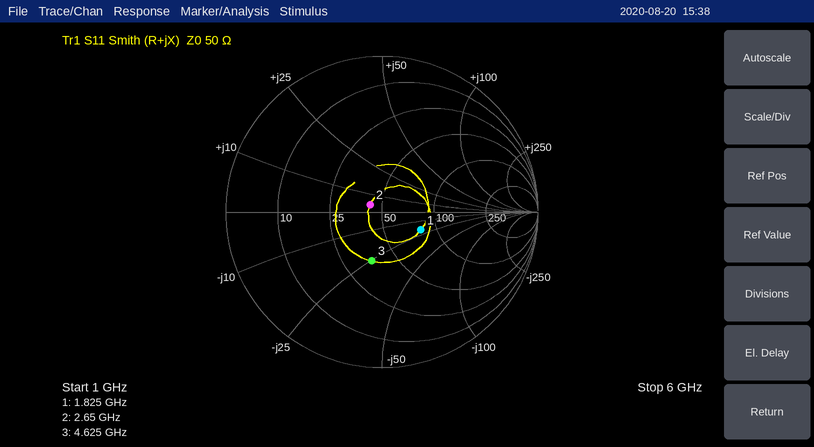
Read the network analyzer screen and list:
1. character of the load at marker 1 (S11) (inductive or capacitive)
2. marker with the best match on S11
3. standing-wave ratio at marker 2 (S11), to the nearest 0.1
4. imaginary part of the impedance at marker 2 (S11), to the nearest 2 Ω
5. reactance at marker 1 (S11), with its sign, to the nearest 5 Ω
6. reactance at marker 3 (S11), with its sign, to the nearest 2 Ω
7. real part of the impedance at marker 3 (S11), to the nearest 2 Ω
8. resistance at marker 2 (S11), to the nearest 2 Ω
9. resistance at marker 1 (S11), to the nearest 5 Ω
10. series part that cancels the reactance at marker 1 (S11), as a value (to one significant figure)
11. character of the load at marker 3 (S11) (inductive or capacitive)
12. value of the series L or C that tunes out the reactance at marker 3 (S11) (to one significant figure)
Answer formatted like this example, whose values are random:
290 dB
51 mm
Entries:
capacitive
marker 2
1.2
+4 Ω
-20 Ω
-26 Ω
36 Ω
42 Ω
80 Ω
2 nH
capacitive
900 pH
